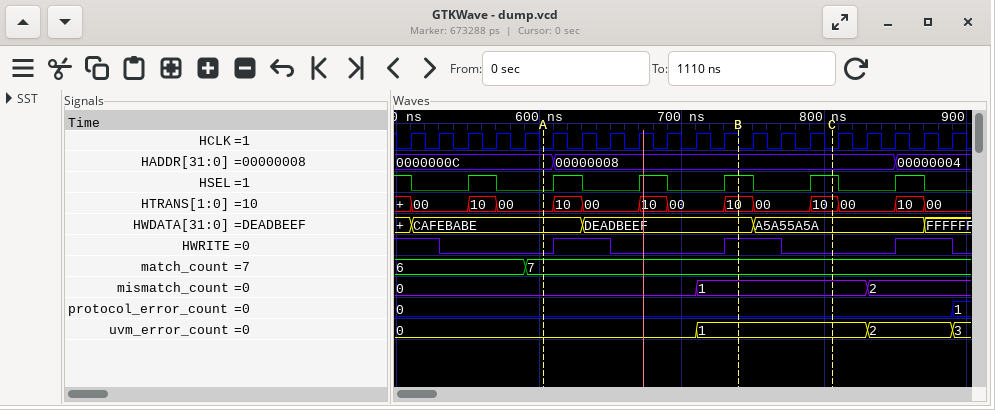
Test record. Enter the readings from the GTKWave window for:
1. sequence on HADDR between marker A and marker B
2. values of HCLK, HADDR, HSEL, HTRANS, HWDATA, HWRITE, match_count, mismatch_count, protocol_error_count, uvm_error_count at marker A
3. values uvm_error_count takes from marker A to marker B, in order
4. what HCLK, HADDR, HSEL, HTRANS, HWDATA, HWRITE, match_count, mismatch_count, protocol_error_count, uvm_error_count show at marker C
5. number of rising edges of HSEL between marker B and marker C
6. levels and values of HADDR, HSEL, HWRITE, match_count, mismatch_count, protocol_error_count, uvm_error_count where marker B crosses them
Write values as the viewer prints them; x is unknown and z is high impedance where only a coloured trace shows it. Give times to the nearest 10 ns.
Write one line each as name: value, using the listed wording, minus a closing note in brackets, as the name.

sequence on HADDR between marker A and marker B: 0000000C, 00000008
values of HCLK, HADDR, HSEL, HTRANS, HWDATA, HWRITE, match_count, mismatch_count, protocol_error_count, uvm_error_count at marker A: HCLK=0, HADDR=0000000C, HSEL=0, HTRANS=00, HWDATA=CAFEBABE, HWRITE=0, match_count=7, mismatch_count=0, protocol_error_count=0, uvm_error_count=0
values uvm_error_count takes from marker A to marker B, in order: 0, 1
what HCLK, HADDR, HSEL, HTRANS, HWDATA, HWRITE, match_count, mismatch_count, protocol_error_count, uvm_error_count show at marker C: HCLK=0, HADDR=00000008, HSEL=1, HTRANS=10, HWDATA=A5A55A5A, HWRITE=0, match_count=7, mismatch_count=1, protocol_error_count=0, uvm_error_count=1
number of rising edges of HSEL between marker B and marker C: 1
levels and values of HADDR, HSEL, HWRITE, match_count, mismatch_count, protocol_error_count, uvm_error_count where marker B crosses them: HADDR=00000008, HSEL=1, HWRITE=1, match_count=7, mismatch_count=1, protocol_error_count=0, uvm_error_count=1
